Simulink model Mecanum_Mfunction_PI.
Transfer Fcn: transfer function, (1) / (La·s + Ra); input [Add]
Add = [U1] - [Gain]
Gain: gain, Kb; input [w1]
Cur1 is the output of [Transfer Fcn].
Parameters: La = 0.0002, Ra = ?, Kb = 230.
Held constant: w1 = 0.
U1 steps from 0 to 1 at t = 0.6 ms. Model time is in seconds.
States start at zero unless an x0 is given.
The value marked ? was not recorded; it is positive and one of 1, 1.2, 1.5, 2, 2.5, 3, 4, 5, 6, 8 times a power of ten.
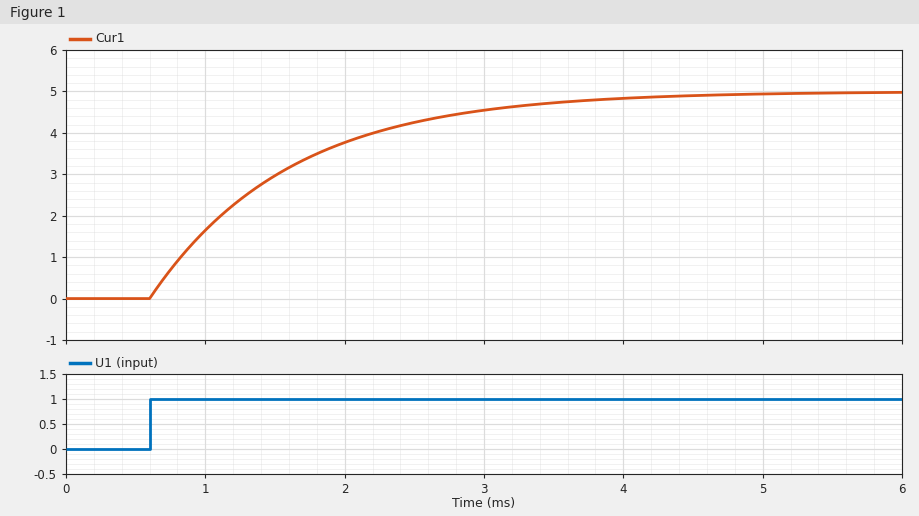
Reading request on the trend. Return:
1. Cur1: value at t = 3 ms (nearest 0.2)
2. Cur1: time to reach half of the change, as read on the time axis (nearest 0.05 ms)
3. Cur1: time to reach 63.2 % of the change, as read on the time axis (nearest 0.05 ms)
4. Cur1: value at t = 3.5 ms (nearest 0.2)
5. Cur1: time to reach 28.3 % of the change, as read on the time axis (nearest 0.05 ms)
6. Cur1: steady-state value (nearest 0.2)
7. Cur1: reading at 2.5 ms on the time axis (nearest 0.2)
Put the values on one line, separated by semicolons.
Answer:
4.6; 1.30 ms; 1.60 ms; 4.8; 0.95 ms; 5.0; 4.2
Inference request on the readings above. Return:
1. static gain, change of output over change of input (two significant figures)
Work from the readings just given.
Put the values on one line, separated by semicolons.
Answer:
5.0
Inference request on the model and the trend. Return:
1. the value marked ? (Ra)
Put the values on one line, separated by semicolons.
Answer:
0.2
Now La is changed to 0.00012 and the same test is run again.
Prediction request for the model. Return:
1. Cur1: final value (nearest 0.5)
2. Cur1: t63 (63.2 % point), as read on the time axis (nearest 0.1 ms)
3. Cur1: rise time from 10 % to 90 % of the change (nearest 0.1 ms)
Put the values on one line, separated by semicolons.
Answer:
5.0; 1.2 ms; 1.3 ms
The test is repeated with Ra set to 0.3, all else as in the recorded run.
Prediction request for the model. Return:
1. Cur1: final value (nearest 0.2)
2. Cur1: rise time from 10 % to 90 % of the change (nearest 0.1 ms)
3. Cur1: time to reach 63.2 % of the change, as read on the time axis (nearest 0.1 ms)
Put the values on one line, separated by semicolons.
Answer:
3.4; 1.5 ms; 1.3 ms
